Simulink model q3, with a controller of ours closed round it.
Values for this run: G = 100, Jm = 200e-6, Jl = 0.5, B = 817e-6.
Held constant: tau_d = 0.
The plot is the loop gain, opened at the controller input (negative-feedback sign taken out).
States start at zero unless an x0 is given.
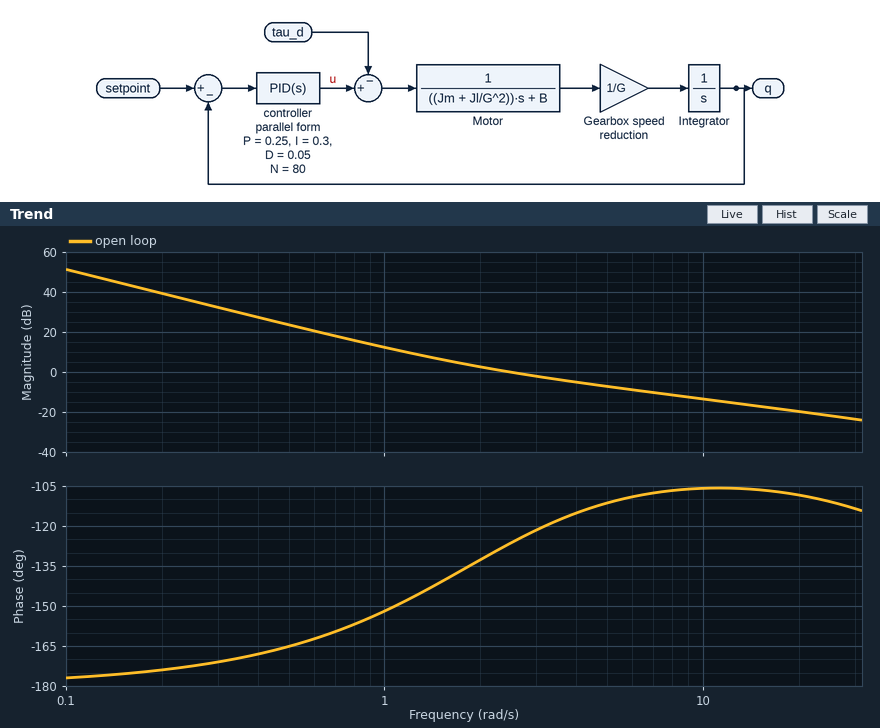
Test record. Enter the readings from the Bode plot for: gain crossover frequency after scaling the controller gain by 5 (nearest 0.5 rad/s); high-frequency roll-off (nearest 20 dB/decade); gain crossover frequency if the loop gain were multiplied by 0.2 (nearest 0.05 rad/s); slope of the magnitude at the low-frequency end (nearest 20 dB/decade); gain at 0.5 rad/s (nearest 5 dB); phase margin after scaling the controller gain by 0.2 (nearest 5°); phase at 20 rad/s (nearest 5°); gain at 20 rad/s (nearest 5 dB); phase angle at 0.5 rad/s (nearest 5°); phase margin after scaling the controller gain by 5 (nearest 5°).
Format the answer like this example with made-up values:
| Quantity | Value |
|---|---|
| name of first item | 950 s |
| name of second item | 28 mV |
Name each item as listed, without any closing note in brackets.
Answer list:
| Quantity | Value |
|---|---|
| gain crossover frequency after scaling the controller gain by 5 | 10.5 rad/s |
| high-frequency roll-off | -20 dB/decade |
| gain crossover frequency if the loop gain were multiplied by 0.2 | 0.90 rad/s |
| slope of the magnitude at the low-frequency end | -40 dB/decade |
| gain at 0.5 rad/s | 25 dB |
| phase margin after scaling the controller gain by 0.2 | 25° |
| phase at 20 rad/s | -110° |
| gain at 20 rad/s | -20 dB |
| phase angle at 0.5 rad/s | -165° |
| phase margin after scaling the controller gain by 5 | 75° |
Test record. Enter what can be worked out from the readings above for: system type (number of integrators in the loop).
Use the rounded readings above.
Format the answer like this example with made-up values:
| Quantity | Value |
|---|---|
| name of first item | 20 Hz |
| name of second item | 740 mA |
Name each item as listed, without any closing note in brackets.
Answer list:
| Quantity | Value |
|---|---|
| system type | 2 |
